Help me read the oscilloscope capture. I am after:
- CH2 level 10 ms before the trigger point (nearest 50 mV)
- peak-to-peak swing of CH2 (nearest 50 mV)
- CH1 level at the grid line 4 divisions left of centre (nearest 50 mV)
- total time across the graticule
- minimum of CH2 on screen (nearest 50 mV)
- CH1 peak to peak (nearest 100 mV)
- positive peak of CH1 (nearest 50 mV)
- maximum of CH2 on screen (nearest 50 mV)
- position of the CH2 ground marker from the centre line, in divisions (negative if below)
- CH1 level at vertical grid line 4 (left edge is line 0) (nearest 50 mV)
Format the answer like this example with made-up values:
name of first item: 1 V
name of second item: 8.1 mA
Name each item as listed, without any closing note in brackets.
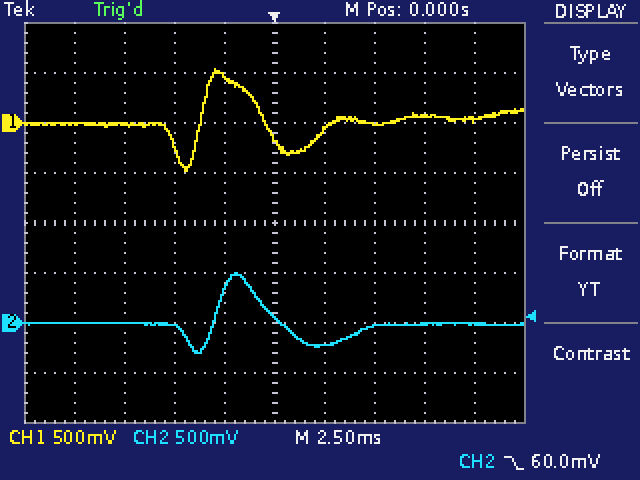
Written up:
CH2 level 10 ms before the trigger point: 0 mV
peak-to-peak swing of CH2: 800 mV
CH1 level at the grid line 4 divisions left of centre: 0 mV
total time across the graticule: 25 ms
minimum of CH2 on screen: -300 mV
CH1 peak to peak: 1.00 V
positive peak of CH1: 550 mV
maximum of CH2 on screen: 500 mV
position of the CH2 ground marker from the centre line, in divisions: -2.0 div
CH1 level at vertical grid line 4 (left edge is line 0): 450 mV
